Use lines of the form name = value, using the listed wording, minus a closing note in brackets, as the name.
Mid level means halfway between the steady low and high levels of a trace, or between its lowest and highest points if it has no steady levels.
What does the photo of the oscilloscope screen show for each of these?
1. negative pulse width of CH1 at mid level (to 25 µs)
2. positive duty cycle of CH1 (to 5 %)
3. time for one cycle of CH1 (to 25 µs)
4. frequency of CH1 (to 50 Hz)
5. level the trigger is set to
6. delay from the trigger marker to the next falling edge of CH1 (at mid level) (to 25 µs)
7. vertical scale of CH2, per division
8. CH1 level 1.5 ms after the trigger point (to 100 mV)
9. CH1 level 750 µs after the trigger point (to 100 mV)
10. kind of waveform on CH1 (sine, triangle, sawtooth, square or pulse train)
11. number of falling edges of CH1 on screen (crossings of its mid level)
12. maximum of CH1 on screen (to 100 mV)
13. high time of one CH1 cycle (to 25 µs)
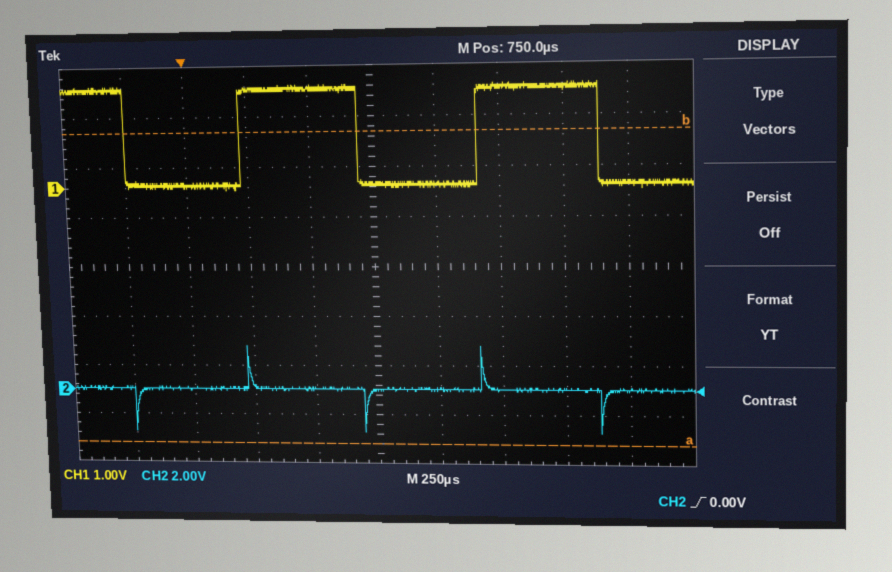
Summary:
negative pulse width of CH1 at mid level = 475 µs
positive duty cycle of CH1 = 50 %
time for one cycle of CH1 = 950 µs
frequency of CH1 = 1.05 kHz
level the trigger is set to = 0.00 V
delay from the trigger marker to the next falling edge of CH1 (at mid level) = 700 µs
vertical scale of CH2, per division = 2 V
CH1 level 1.5 ms after the trigger point = 1.9 V
CH1 level 750 µs after the trigger point = 100 mV
kind of waveform on CH1 = square
number of falling edges of CH1 on screen = 3
maximum of CH1 on screen = 2.0 V
high time of one CH1 cycle = 475 µs
